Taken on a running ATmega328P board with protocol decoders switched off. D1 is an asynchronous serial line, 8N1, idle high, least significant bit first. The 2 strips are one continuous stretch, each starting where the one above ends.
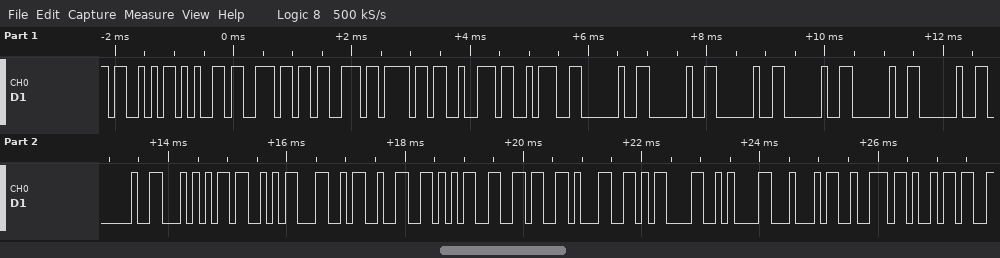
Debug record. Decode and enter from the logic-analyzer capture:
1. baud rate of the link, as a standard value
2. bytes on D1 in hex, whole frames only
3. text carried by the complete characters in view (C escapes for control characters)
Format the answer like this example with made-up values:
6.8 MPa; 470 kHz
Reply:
9600 baud; 53 65 6E 73 6F 72 3A 20 20 20 20 20 20 20 54 53 4C 32 35 36 31 0D 0A 44 72 69; "Sensor:       TSL2561\r\nDri"
